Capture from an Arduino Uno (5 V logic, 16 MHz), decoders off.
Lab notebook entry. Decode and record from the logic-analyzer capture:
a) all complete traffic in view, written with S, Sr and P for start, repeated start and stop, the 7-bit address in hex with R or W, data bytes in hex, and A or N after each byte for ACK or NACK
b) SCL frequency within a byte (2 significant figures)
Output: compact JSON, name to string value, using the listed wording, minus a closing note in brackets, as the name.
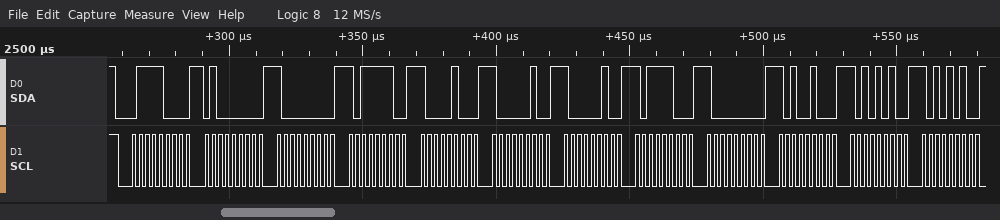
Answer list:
{"all complete traffic in view, written with S, Sr and P for start, repeated start and stop, the 7-bit address in hex with R or W, data bytes in hex, and A or N after each byte for ACK or NACK": "S 3CW A 40 A 80 A BE A 84 A 82 A 82 A BC A 80 A A4 A AA A AA A", "SCL frequency within a byte": "400 kHz"}
